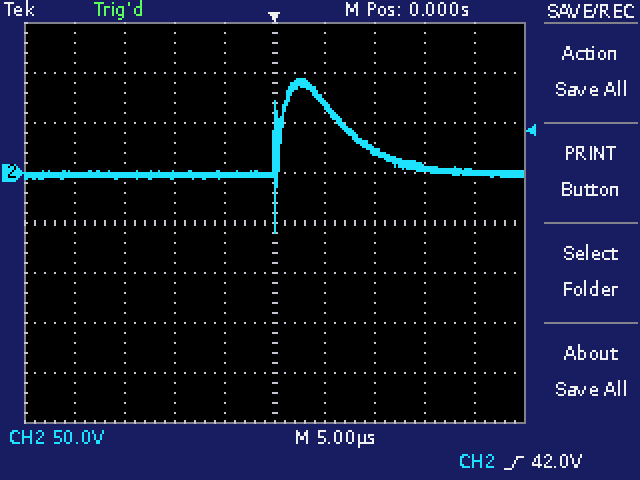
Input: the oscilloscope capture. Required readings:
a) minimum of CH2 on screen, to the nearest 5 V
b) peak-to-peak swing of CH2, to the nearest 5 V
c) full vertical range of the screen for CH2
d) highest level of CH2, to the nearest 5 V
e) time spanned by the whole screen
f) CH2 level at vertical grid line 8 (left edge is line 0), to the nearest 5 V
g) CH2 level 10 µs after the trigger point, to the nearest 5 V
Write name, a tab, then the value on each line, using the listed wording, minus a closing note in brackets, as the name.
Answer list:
minimum of CH2 on screen, to the nearest 5 V	-60 V
peak-to-peak swing of CH2, to the nearest 5 V	155 V
full vertical range of the screen for CH2	400 V
highest level of CH2, to the nearest 5 V	95 V
time spanned by the whole screen	50 µs
CH2 level at vertical grid line 8 (left edge is line 0), to the nearest 5 V	5 V
CH2 level 10 µs after the trigger point, to the nearest 5 V	25 V
